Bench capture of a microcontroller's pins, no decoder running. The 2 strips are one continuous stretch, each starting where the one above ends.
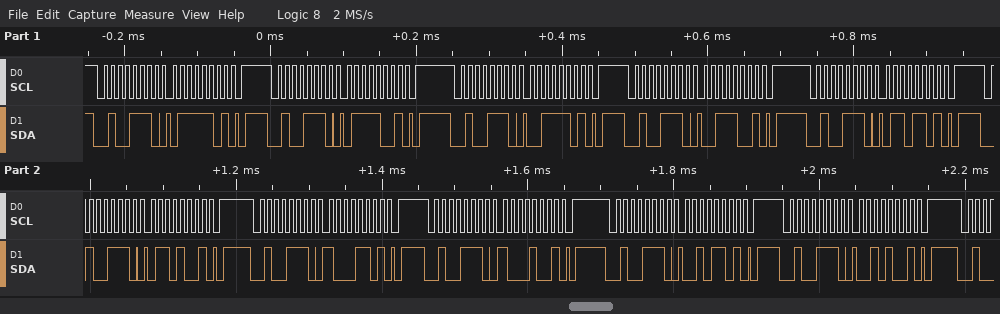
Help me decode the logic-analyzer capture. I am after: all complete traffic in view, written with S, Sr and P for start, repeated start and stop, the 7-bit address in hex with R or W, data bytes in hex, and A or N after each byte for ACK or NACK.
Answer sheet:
S 27W A 7D A P S 27W A 79 A P S 27W A 3D A P S 27W A 39 A P S 27W A 6D A P S 27W A 69 A P S 27W A 8D A P S 27W A 89 A P S 27W A 2D A P S 27W A 29 A P
